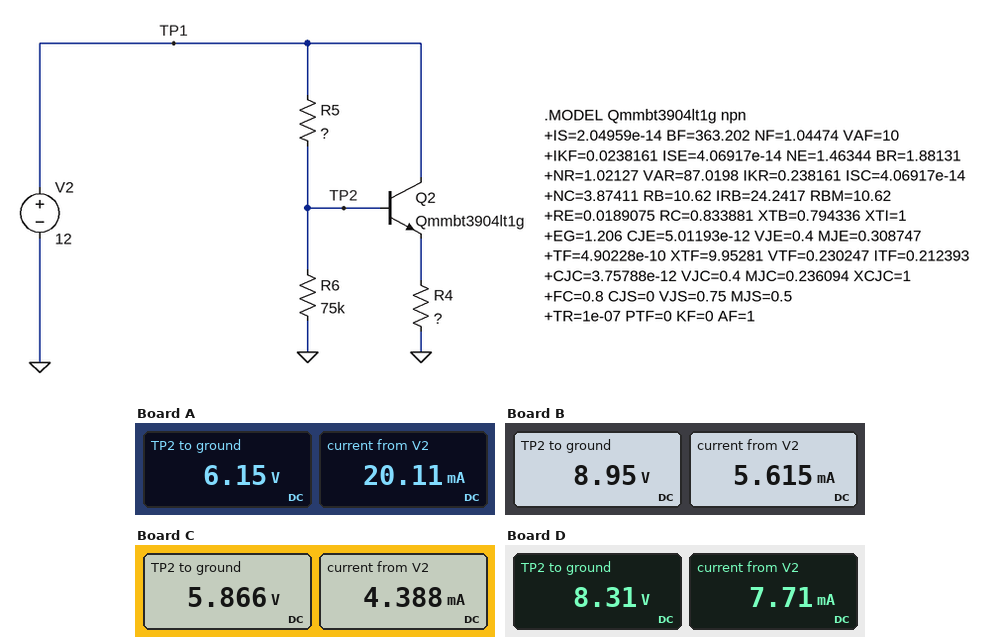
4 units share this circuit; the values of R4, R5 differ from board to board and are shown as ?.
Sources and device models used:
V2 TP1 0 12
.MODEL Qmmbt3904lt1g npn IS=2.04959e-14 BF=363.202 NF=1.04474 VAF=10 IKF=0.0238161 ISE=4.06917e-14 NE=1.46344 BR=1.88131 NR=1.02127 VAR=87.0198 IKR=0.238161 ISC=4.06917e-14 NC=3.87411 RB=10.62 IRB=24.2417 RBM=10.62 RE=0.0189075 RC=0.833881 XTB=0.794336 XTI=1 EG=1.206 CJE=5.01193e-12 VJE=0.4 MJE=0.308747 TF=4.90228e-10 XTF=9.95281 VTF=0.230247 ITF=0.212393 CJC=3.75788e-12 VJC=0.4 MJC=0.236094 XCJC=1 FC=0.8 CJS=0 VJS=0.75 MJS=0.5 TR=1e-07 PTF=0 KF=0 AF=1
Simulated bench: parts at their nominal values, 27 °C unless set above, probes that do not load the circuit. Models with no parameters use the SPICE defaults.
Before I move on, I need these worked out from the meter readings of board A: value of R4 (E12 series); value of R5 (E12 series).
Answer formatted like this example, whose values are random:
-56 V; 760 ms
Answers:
270 Ω; 39 kΩ
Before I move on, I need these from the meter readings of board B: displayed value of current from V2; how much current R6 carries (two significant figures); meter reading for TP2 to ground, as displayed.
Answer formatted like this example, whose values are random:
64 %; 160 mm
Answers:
5.615 mA; 120 µA; 8.95 V
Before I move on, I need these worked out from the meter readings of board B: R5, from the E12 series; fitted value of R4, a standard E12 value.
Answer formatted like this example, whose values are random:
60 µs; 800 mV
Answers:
22 kΩ; 1.5 kΩ
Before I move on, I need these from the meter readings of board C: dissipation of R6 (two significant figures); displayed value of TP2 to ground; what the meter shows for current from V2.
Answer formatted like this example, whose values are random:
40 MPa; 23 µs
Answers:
460 µW; 5.866 V; 4.388 mA
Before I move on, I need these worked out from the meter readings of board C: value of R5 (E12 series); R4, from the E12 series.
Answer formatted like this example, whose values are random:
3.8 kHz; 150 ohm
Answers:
68 kΩ; 1.2 kΩ
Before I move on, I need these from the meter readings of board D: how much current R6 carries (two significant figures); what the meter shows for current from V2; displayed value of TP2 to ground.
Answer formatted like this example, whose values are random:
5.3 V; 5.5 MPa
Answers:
110 µA; 7.71 mA; 8.31 V
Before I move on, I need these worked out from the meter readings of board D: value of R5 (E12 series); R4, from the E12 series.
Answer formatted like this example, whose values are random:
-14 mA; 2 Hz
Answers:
27 kΩ; 1 kΩ
